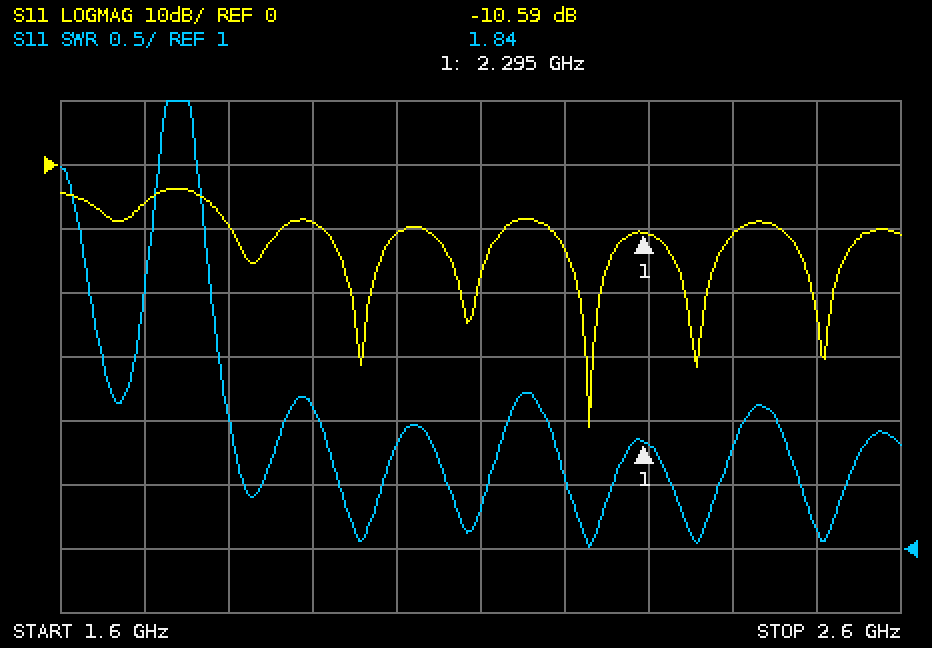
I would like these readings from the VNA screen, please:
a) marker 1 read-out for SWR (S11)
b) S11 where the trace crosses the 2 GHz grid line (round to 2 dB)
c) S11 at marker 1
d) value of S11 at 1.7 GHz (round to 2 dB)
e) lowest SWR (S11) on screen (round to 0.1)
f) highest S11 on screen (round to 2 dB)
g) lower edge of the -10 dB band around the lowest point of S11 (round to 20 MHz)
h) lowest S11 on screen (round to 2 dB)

1.84
-10 dB
-10.59 dB
-6 dB
1.0
-4 dB
2.18 GHz
-40 dB
